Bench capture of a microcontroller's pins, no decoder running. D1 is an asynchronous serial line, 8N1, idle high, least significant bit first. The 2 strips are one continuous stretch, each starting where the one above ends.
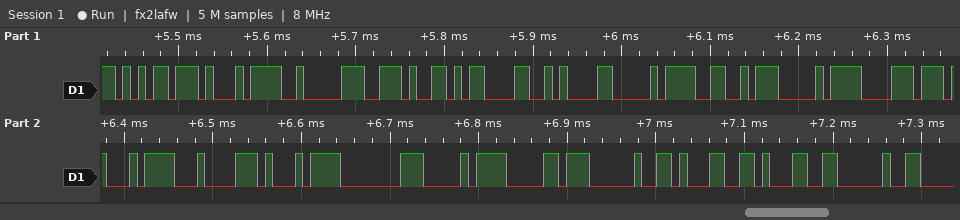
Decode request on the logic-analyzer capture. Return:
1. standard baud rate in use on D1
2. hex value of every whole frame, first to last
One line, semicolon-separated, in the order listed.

115200 baud; B5 D1 82 2E 0D 0A D0 A6 D0 B8 D1 84 D1 80 D0 B0 20 31 31 20
